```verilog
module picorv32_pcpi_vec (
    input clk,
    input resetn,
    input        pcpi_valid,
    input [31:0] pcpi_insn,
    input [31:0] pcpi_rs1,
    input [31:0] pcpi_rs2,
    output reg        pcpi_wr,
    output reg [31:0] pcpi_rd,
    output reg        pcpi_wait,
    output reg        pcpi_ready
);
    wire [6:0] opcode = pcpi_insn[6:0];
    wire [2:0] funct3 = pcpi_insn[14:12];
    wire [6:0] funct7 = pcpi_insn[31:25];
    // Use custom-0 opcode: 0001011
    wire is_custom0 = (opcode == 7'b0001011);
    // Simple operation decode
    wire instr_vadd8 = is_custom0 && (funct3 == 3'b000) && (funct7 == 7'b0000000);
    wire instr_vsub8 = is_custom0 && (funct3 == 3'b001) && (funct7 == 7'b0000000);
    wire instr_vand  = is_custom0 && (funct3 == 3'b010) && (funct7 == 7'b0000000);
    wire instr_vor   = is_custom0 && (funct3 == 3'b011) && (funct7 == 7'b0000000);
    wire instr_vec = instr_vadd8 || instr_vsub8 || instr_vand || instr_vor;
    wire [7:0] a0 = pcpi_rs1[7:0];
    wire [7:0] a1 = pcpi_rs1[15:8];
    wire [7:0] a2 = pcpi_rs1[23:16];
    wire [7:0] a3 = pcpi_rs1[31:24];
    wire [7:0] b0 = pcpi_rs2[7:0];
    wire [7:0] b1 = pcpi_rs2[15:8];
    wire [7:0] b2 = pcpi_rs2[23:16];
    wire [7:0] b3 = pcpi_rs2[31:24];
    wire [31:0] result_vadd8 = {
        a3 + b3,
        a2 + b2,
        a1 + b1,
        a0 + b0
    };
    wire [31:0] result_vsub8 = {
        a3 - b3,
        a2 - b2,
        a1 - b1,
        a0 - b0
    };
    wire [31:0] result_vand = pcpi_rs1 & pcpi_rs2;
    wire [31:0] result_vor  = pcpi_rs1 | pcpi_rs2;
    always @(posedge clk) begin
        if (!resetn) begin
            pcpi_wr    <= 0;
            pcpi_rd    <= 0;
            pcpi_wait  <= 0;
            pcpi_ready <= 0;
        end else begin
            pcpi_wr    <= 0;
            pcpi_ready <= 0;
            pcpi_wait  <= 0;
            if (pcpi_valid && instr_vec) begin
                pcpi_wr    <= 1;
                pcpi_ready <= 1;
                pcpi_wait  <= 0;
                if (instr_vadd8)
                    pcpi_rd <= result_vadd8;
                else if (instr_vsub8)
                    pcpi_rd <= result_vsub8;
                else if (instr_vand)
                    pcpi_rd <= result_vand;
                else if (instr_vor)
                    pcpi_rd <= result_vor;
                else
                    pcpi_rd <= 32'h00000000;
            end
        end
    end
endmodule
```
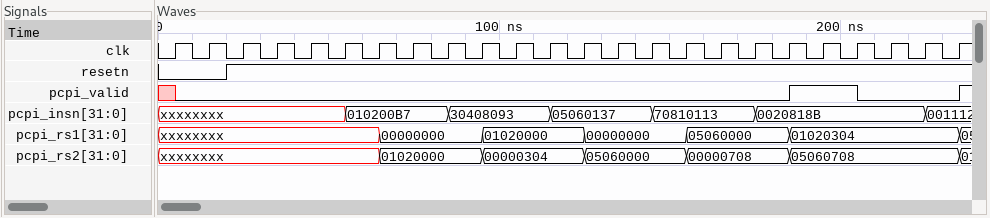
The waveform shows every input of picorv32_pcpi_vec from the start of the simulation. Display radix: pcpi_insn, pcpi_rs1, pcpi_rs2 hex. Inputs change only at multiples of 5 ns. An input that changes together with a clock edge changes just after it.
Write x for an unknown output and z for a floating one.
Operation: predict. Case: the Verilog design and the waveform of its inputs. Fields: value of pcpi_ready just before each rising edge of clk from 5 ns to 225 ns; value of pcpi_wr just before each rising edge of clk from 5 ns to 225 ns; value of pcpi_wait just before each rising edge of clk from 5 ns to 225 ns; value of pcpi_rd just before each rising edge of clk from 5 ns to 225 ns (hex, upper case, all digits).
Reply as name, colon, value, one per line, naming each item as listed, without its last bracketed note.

value of pcpi_ready just before each rising edge of clk from 5 ns to 225 ns: x 0 0 0 0 0 0 0 0 0 0 0 0 0 0 0 0 0 0 0 1 1 0
value of pcpi_wr just before each rising edge of clk from 5 ns to 225 ns: x 0 0 0 0 0 0 0 0 0 0 0 0 0 0 0 0 0 0 0 1 1 0
value of pcpi_wait just before each rising edge of clk from 5 ns to 225 ns: x 0 0 0 0 0 0 0 0 0 0 0 0 0 0 0 0 0 0 0 0 0 0
value of pcpi_rd just before each rising edge of clk from 5 ns to 225 ns: x, 00000000, 00000000, 00000000, 00000000, 00000000, 00000000, 00000000, 00000000, 00000000, 00000000, 00000000, 00000000, 00000000, 00000000, 00000000, 00000000, 00000000, 00000000, 00000000, 06080A0C, 06080A0C, 06080A0C
